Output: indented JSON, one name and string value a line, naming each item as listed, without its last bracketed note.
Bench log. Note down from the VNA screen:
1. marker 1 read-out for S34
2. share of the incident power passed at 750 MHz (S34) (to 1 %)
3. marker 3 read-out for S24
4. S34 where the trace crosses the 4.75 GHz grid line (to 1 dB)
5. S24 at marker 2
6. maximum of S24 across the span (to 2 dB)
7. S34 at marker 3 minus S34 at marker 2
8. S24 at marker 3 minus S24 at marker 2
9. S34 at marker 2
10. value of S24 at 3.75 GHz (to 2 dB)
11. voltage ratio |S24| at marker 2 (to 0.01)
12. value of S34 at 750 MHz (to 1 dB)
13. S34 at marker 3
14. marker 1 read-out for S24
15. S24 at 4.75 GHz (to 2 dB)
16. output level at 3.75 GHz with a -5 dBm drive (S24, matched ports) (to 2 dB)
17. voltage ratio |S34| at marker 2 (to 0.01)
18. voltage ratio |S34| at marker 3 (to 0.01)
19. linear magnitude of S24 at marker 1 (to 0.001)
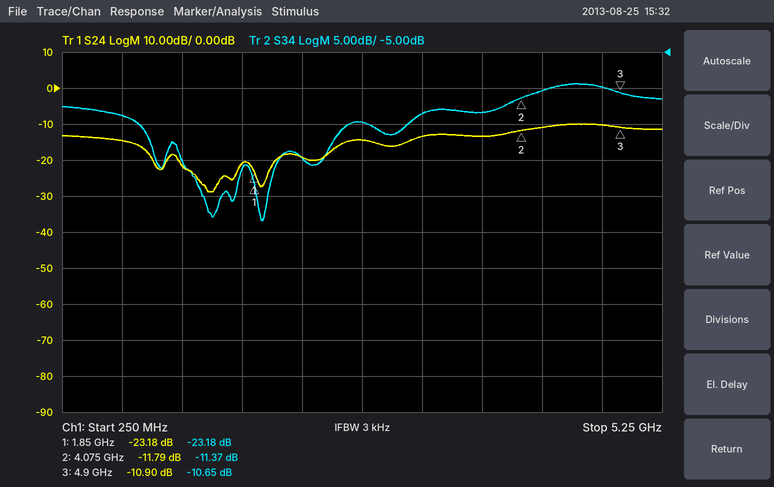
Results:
{
  "marker 1 read-out for S34": "-23.18 dB",
  "share of the incident power passed at 750 MHz (S34)": "4 %",
  "marker 3 read-out for S24": "-10.90 dB",
  "S34 where the trace crosses the 4.75 GHz grid line": "-10 dB",
  "S24 at marker 2": "-11.79 dB",
  "maximum of S24 across the span": "-10 dB",
  "S34 at marker 3 minus S34 at marker 2": "0.72 dB",
  "S24 at marker 3 minus S24 at marker 2": "0.89 dB",
  "S34 at marker 2": "-11.37 dB",
  "value of S24 at 3.75 GHz": "-14 dB",
  "voltage ratio |S24| at marker 2": "0.26",
  "value of S34 at 750 MHz": "-14 dB",
  "S34 at marker 3": "-10.65 dB",
  "marker 1 read-out for S24": "-23.18 dB",
  "S24 at 4.75 GHz": "-10 dB",
  "output level at 3.75 GHz with a -5 dBm drive (S24, matched ports)": "-18 dBm",
  "voltage ratio |S34| at marker 2": "0.27",
  "voltage ratio |S34| at marker 3": "0.29",
  "linear magnitude of S24 at marker 1": "0.069"
}
